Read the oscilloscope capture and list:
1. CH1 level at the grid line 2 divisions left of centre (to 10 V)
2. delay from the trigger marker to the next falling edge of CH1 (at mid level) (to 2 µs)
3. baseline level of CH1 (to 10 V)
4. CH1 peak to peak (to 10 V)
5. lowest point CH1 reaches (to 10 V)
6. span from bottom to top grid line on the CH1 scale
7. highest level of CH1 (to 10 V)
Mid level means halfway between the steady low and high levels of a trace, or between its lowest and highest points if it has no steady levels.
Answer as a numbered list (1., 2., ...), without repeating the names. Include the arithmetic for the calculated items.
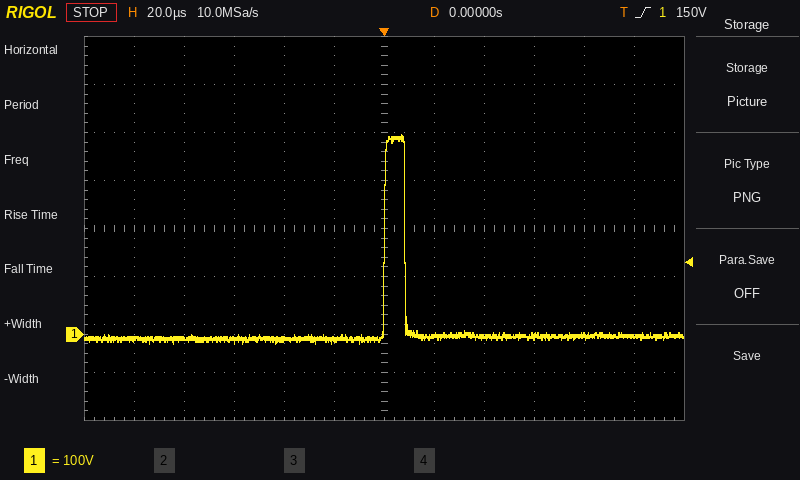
1. -10 V
2. 8 µs
3. -10 V
4. 420 V − (-20 V) = 440 V
5. -20 V
6. 800 V
7. 420 V
